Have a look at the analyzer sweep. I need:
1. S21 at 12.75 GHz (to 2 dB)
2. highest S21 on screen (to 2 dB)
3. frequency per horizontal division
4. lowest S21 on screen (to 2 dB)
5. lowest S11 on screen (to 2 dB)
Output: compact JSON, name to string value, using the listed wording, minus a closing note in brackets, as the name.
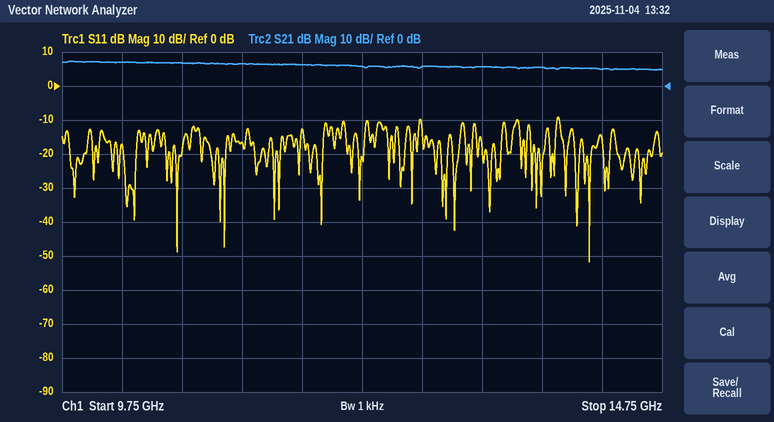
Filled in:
{"S21 at 12.75 GHz": "6 dB", "highest S21 on screen": "8 dB", "frequency per horizontal division": "500 MHz", "lowest S21 on screen": "4 dB", "lowest S11 on screen": "-52 dB"}
